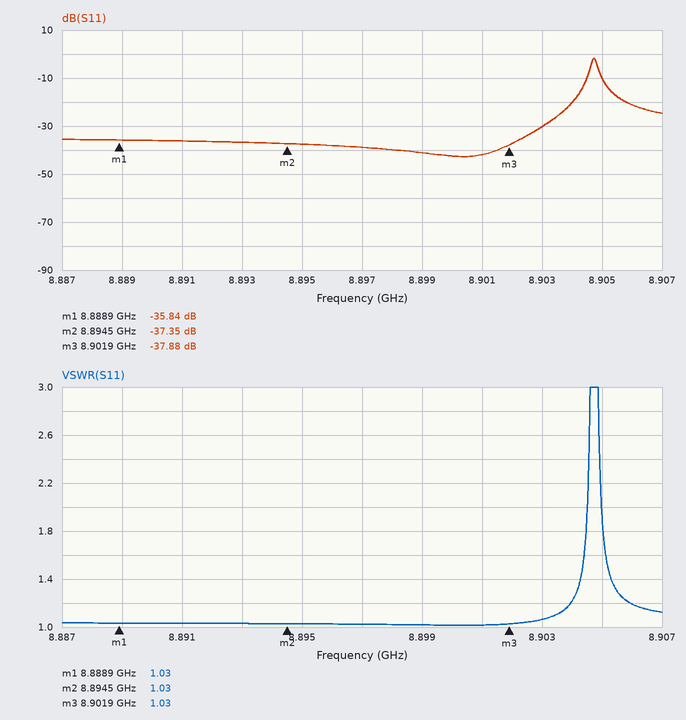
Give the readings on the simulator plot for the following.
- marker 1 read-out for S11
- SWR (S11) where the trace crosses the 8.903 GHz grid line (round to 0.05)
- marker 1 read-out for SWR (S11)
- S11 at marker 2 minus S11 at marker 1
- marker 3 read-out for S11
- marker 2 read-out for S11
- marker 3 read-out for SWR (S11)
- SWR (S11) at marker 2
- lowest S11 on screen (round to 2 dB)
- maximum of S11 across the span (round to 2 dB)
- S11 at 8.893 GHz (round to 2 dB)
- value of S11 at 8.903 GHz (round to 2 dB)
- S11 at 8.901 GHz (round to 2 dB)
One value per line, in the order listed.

-35.84 dB
1.05
1.03
-1.51 dB
-37.88 dB
-37.35 dB
1.03
1.03
-42 dB
-2 dB
-36 dB
-30 dB
-42 dB
